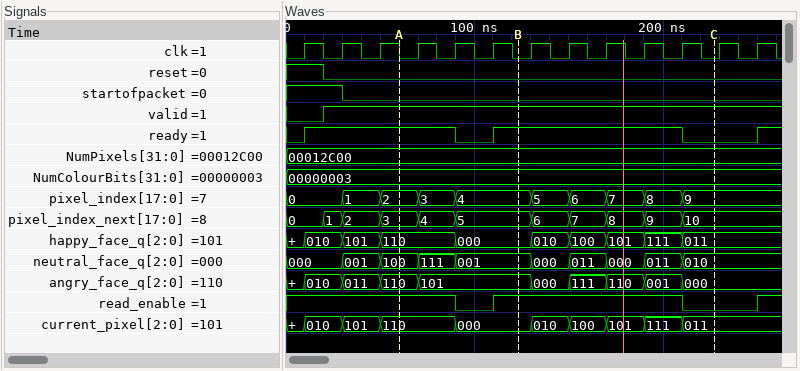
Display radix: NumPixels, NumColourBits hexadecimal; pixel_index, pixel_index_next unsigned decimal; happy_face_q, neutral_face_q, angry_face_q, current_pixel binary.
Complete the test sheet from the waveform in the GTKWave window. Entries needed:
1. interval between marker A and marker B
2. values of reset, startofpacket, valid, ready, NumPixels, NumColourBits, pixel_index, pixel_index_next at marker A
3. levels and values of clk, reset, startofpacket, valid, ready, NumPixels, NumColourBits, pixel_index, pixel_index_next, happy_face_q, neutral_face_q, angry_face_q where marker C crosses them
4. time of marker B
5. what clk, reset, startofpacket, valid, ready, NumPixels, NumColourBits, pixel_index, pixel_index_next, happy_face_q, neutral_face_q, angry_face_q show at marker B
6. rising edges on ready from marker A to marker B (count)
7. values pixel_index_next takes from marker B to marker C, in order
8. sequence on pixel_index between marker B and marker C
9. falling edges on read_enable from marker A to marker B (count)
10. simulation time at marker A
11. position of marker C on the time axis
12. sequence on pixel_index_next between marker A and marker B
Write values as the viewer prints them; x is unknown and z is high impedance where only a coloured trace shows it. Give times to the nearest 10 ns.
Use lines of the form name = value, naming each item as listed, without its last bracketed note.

interval between marker A and marker B = 60 ns
values of reset, startofpacket, valid, ready, NumPixels, NumColourBits, pixel_index, pixel_index_next at marker A = reset=0, startofpacket=0, valid=1, ready=1, NumPixels=00012C00, NumColourBits=00000003, pixel_index=2, pixel_index_next=3
levels and values of clk, reset, startofpacket, valid, ready, NumPixels, NumColourBits, pixel_index, pixel_index_next, happy_face_q, neutral_face_q, angry_face_q where marker C crosses them = clk=0, reset=0, startofpacket=0, valid=1, ready=0, NumPixels=00012C00, NumColourBits=00000003, pixel_index=9, pixel_index_next=10, happy_face_q=011, neutral_face_q=010, angry_face_q=000
time of marker B = 120 ns
what clk, reset, startofpacket, valid, ready, NumPixels, NumColourBits, pixel_index, pixel_index_next, happy_face_q, neutral_face_q, angry_face_q show at marker B = clk=0, reset=0, startofpacket=0, valid=1, ready=1, NumPixels=00012C00, NumColourBits=00000003, pixel_index=4, pixel_index_next=5, happy_face_q=000, neutral_face_q=001, angry_face_q=101
rising edges on ready from marker A to marker B = 1
values pixel_index_next takes from marker B to marker C, in order = 5, 6, 7, 8, 9, 10
sequence on pixel_index between marker B and marker C = 4, 5, 6, 7, 8, 9
falling edges on read_enable from marker A to marker B = 1
simulation time at marker A = 60 ns
position of marker C on the time axis = 230 ns
sequence on pixel_index_next between marker A and marker B = 3, 4, 5
